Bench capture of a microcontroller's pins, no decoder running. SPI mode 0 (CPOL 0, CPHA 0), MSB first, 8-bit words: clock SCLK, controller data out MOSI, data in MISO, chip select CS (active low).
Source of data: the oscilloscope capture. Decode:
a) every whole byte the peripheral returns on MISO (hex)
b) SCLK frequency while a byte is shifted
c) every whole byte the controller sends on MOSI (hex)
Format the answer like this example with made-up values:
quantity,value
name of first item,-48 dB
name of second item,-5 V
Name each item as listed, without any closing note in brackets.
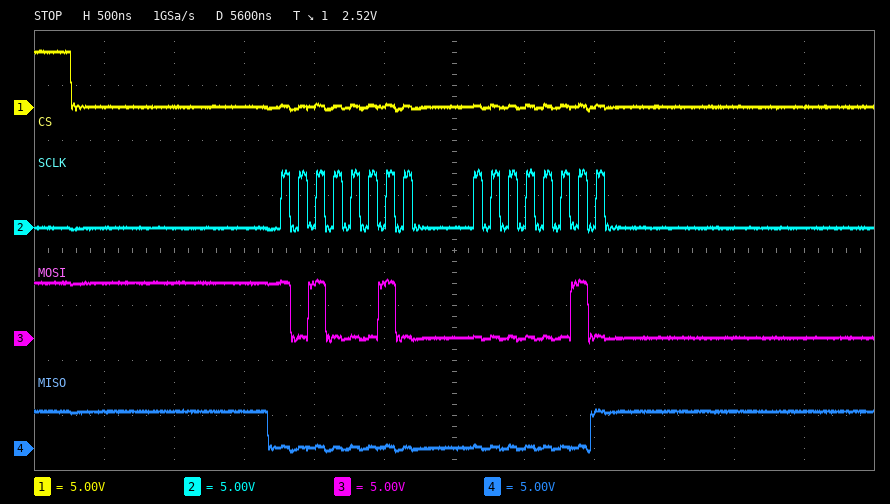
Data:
quantity,value
every whole byte the peripheral returns on MISO,0x00 0x01
SCLK frequency while a byte is shifted,8 MHz
every whole byte the controller sends on MOSI,0xA2 0x02
